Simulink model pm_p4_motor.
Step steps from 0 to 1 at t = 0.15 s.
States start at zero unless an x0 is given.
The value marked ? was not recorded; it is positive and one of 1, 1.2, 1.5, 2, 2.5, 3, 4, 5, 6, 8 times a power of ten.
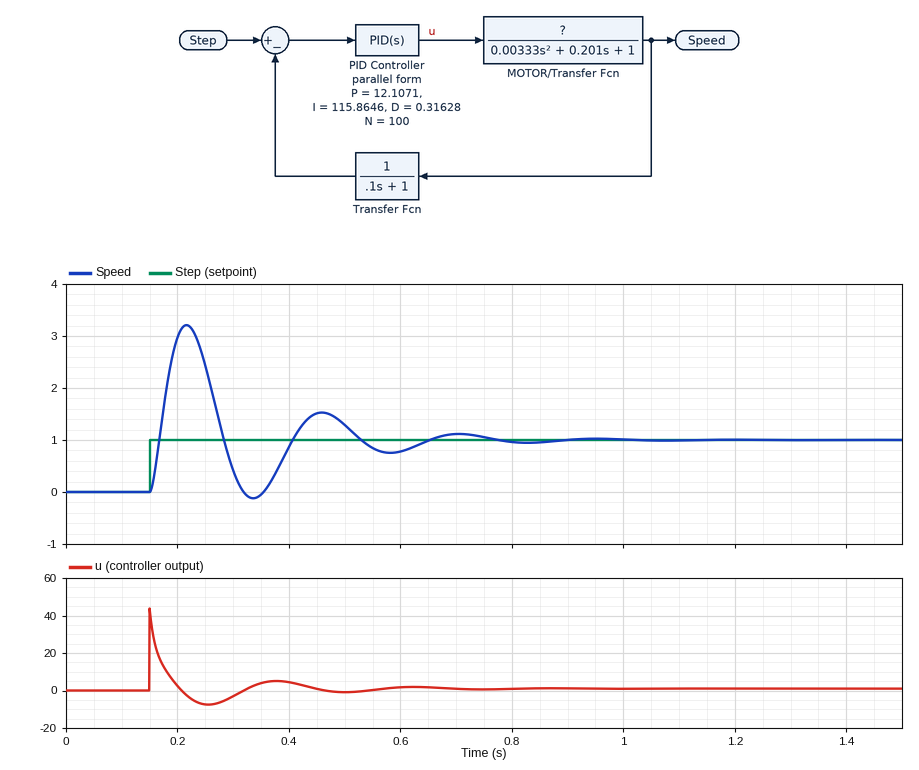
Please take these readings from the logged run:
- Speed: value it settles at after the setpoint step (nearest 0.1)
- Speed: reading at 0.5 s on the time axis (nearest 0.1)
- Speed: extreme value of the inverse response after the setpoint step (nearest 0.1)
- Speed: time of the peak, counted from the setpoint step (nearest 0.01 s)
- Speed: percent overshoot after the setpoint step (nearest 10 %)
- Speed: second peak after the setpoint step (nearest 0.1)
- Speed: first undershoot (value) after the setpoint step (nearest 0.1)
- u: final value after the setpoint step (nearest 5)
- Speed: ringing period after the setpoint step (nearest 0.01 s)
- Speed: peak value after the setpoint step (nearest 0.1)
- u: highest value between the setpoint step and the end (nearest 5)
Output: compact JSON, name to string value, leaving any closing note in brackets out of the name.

{"Speed: value it settles at after the setpoint step": "1.0", "Speed: reading at 0.5 s on the time axis": "1.3", "Speed: extreme value of the inverse response after the setpoint step": "-0.1", "Speed: time of the peak, counted from the setpoint step": "0.07 s", "Speed: percent overshoot after the setpoint step": "220 %", "Speed: second peak after the setpoint step": "1.5", "Speed: first undershoot (value) after the setpoint step": "-0.1", "u: final value after the setpoint step": "0", "Speed: ringing period after the setpoint step": "0.24 s", "Speed: peak value after the setpoint step": "3.2", "u: highest value between the setpoint step and the end": "45"}
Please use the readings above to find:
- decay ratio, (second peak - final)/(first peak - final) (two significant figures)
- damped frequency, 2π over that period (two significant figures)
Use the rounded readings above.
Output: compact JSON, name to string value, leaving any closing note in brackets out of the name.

{"decay ratio, (second peak - final)/(first peak - final)": "0.23", "damped frequency, 2π over that period": "26 rad/s"}
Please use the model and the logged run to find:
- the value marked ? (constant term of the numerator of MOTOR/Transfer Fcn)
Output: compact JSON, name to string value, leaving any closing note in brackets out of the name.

{"the value marked ?": "1"}
